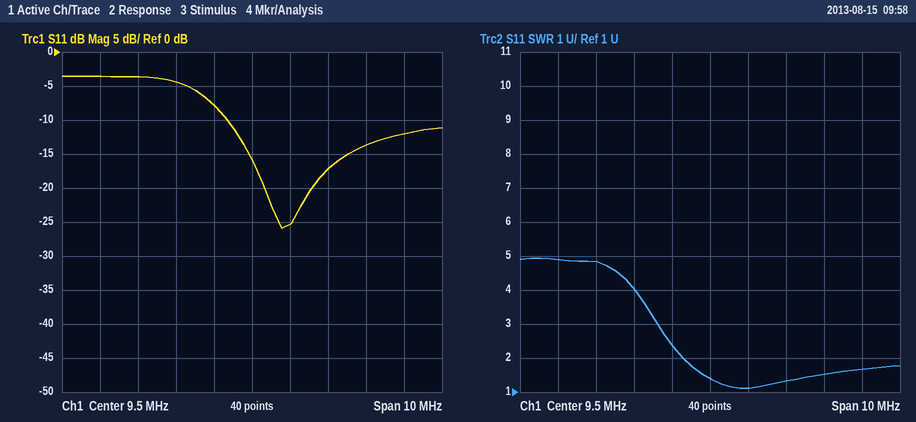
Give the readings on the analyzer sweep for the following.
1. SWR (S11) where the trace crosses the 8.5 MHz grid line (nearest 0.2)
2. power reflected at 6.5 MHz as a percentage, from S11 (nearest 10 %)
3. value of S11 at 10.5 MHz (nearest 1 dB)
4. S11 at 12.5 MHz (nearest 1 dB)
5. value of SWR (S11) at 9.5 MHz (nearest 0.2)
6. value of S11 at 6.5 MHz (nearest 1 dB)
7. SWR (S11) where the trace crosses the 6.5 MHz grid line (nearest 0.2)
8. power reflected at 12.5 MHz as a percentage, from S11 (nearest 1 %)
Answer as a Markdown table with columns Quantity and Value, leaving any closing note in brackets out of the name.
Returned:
| Quantity | Value |
|---|---|
| SWR (S11) where the trace crosses the 8.5 MHz grid line | 2.4 |
| power reflected at 6.5 MHz as a percentage, from S11 | 40 % |
| value of S11 at 10.5 MHz | -25 dB |
| S11 at 12.5 MHz | -14 dB |
| value of SWR (S11) at 9.5 MHz | 1.4 |
| value of S11 at 6.5 MHz | -4 dB |
| SWR (S11) where the trace crosses the 6.5 MHz grid line | 4.8 |
| power reflected at 12.5 MHz as a percentage, from S11 | 4 % |
